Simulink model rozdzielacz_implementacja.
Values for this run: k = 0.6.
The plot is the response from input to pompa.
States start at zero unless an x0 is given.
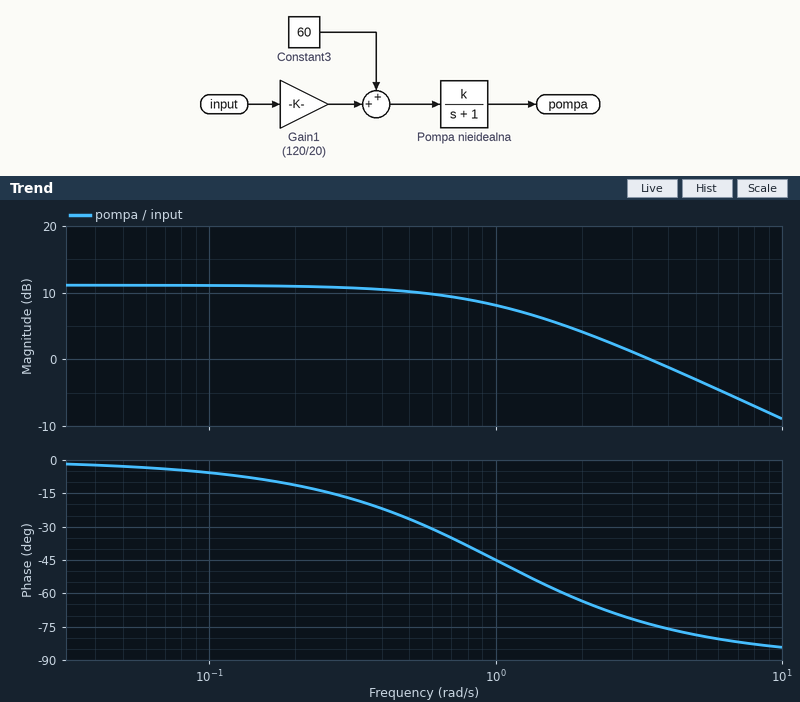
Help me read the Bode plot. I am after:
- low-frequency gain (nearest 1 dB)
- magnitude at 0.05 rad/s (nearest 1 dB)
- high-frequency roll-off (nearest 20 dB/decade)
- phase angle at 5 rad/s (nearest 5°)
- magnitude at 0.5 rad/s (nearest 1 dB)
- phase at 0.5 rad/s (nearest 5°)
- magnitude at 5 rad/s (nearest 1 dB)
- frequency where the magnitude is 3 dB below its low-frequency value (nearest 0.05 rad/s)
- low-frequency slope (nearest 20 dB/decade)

11 dB
11 dB
-20 dB/decade
-80°
10 dB
-25°
-3 dB
1.00 rad/s
0 dB/decade
